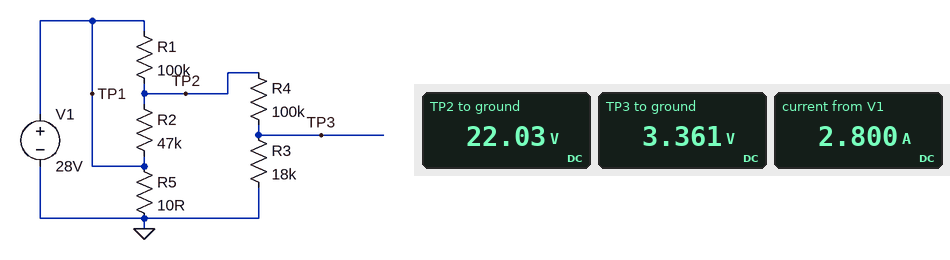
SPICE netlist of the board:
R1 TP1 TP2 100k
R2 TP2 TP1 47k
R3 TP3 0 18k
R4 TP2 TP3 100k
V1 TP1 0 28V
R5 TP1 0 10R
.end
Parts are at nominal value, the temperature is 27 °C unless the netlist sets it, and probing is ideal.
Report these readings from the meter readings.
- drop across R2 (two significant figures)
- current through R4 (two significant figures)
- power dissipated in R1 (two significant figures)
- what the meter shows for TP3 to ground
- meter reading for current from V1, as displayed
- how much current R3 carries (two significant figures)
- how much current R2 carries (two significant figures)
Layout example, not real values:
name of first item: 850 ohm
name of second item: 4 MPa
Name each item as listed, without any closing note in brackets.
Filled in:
drop across R2: 6.0 V
current through R4: 190 µA
power dissipated in R1: 360 µW
what the meter shows for TP3 to ground: 3.361 V
meter reading for current from V1, as displayed: 2.800 A
how much current R3 carries: 190 µA
how much current R2 carries: 130 µA
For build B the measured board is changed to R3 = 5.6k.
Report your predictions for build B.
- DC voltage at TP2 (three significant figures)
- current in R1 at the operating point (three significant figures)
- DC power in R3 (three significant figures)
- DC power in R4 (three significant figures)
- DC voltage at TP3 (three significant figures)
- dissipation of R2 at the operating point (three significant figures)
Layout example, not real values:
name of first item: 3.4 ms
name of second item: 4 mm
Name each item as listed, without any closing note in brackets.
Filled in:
DC voltage at TP2: 21.5 V
current in R1 at the operating point: 65.1 µA
DC power in R3: 232 µW
DC power in R4: 4.14 mW
DC voltage at TP3: 1.14 V
dissipation of R2 at the operating point: 901 µW
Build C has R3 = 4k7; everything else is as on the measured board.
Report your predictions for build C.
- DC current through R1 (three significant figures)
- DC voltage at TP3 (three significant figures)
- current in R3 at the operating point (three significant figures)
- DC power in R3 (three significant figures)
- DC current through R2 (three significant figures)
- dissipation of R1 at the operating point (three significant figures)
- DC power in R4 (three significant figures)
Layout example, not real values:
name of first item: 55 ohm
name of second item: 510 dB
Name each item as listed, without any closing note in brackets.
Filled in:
DC current through R1: 65.5 µA
DC voltage at TP3: 963 mV
current in R3 at the operating point: 205 µA
DC power in R3: 197 µW
DC current through R2: 139 µA
dissipation of R1 at the operating point: 429 µW
DC power in R4: 4.20 mW
